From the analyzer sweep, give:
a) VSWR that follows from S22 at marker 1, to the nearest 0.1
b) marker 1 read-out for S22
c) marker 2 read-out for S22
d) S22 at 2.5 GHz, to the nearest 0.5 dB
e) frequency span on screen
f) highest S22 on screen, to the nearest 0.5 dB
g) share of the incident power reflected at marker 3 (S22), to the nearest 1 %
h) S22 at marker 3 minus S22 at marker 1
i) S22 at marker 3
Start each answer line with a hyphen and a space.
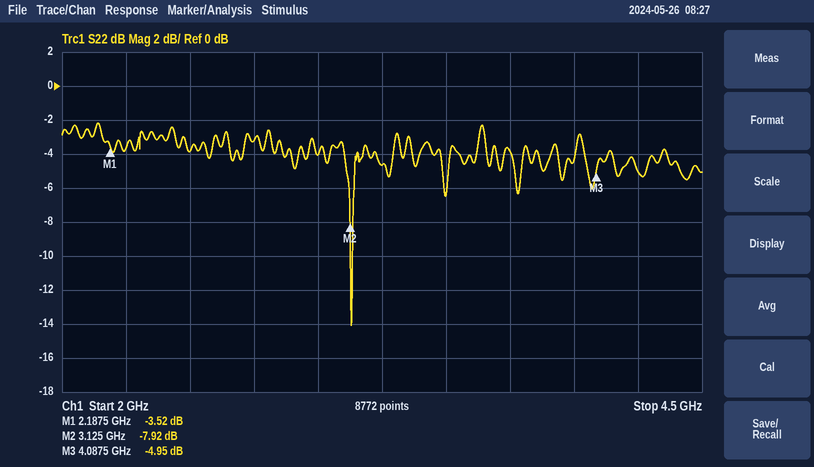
- 5.0
- -3.52 dB
- -7.92 dB
- -4.0 dB
- 2.5 GHz
- -2.0 dB
- 32 %
- -1.43 dB
- -4.95 dB
